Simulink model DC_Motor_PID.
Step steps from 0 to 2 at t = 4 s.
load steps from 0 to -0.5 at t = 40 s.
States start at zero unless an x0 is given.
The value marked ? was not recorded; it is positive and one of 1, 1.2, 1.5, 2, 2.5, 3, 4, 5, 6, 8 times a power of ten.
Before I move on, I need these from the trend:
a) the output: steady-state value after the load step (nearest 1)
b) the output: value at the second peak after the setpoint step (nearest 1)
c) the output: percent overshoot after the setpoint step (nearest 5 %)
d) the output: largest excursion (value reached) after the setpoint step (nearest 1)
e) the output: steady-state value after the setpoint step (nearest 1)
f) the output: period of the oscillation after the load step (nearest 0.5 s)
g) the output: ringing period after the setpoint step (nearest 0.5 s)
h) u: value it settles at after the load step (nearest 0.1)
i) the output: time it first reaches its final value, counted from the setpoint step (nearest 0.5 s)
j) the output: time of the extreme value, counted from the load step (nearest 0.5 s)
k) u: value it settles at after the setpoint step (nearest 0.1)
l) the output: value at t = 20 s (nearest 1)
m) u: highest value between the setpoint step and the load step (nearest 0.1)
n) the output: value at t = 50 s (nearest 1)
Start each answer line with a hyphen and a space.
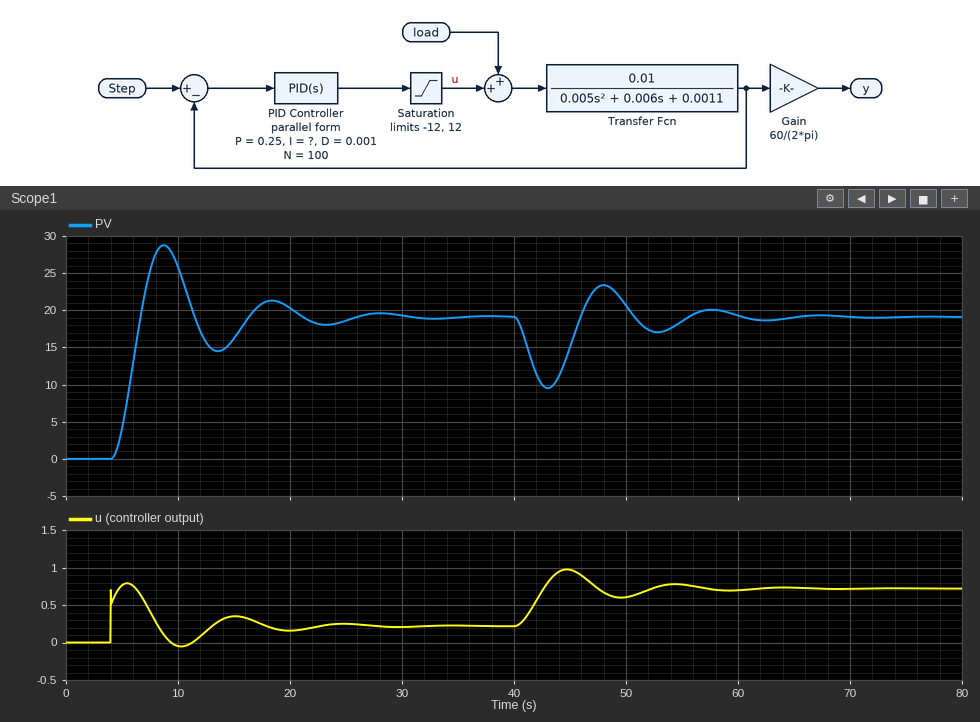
- 19
- 21
- 50 %
- 29
- 19
- 10.0 s
- 9.5 s
- 0.7
- 2.5 s
- 3.0 s
- 0.2
- 20
- 0.8
- 21
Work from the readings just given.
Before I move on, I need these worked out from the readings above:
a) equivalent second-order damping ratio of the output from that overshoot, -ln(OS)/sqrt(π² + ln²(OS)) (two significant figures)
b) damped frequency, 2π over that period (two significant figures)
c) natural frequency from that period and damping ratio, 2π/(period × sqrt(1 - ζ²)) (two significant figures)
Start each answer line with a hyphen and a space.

- 0.22
- 0.66 rad/s
- 0.68 rad/s
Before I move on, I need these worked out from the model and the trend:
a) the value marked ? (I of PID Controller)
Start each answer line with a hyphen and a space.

- 0.2
